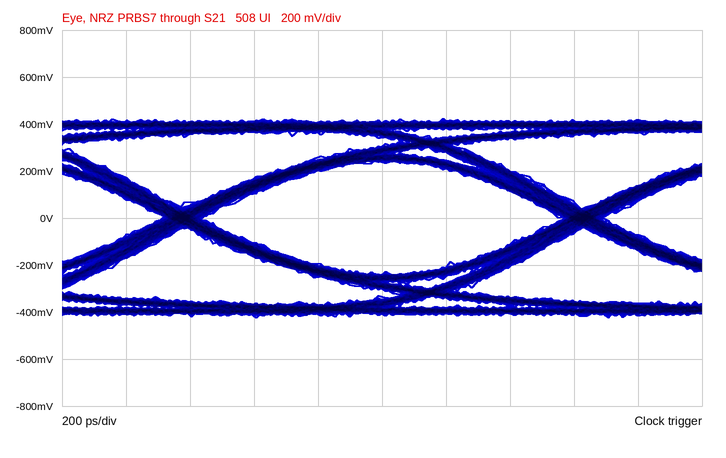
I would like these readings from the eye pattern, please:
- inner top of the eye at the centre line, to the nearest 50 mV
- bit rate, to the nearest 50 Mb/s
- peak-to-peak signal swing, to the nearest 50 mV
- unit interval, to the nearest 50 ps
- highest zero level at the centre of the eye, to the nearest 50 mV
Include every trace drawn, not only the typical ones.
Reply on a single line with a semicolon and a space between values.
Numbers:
250 mV; 800 Mb/s; 850 mV; 1.25 ns; -250 mV
